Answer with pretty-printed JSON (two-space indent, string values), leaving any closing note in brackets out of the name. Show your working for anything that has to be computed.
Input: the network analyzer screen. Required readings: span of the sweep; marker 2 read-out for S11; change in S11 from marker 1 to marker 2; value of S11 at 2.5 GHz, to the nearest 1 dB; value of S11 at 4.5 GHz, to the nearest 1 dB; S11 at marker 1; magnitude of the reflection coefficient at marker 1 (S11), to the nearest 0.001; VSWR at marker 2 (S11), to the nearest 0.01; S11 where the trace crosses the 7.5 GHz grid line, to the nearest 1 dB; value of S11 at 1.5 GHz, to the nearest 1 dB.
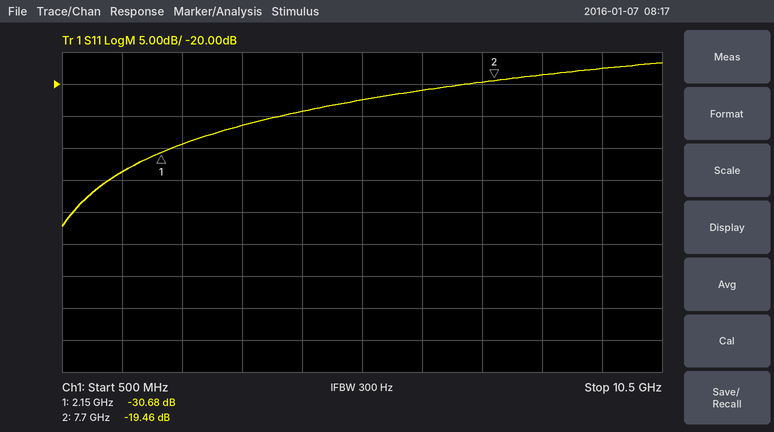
{
  "span of the sweep": "10 GHz",
  "marker 2 read-out for S11": "-19.46 dB",
  "change in S11 from marker 1 to marker 2": "-19.46 − (-30.68) = 11.22 dB",
  "value of S11 at 2.5 GHz, to the nearest 1 dB": "-29 dB",
  "value of S11 at 4.5 GHz, to the nearest 1 dB": "-24 dB",
  "S11 at marker 1": "-30.68 dB",
  "magnitude of the reflection coefficient at marker 1 (S11), to the nearest 0.001": "10^(-30.68/20) ≈ 0.029",
  "VSWR at marker 2 (S11), to the nearest 0.01": "(1 + 0.1064)/(1 − 0.1064) ≈ 1.24",
  "S11 where the trace crosses the 7.5 GHz grid line, to the nearest 1 dB": "-20 dB",
  "value of S11 at 1.5 GHz, to the nearest 1 dB": "-34 dB"
}
